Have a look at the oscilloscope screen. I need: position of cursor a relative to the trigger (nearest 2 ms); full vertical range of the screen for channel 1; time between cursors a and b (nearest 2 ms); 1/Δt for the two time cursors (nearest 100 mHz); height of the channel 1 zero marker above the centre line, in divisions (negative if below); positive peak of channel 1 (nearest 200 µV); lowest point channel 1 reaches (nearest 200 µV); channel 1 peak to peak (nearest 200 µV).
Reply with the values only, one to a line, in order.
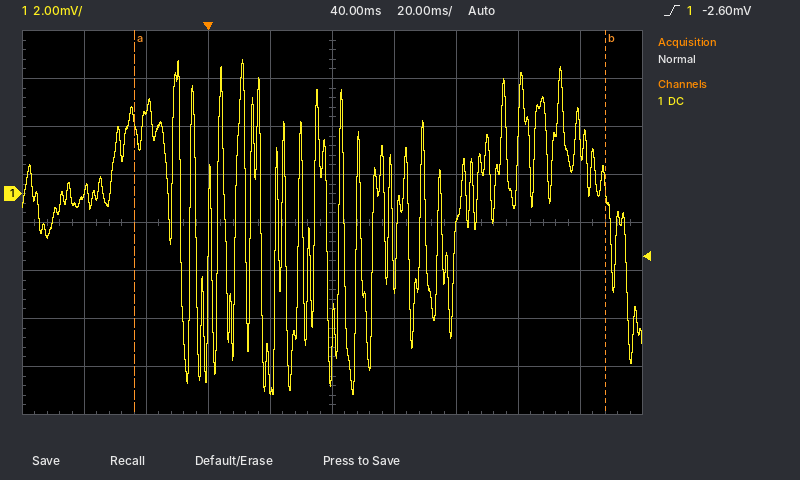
-24 ms
16 mV
152 ms
6.6 Hz
+0.6 div
5.6 mV
-8.4 mV
14.0 mV
